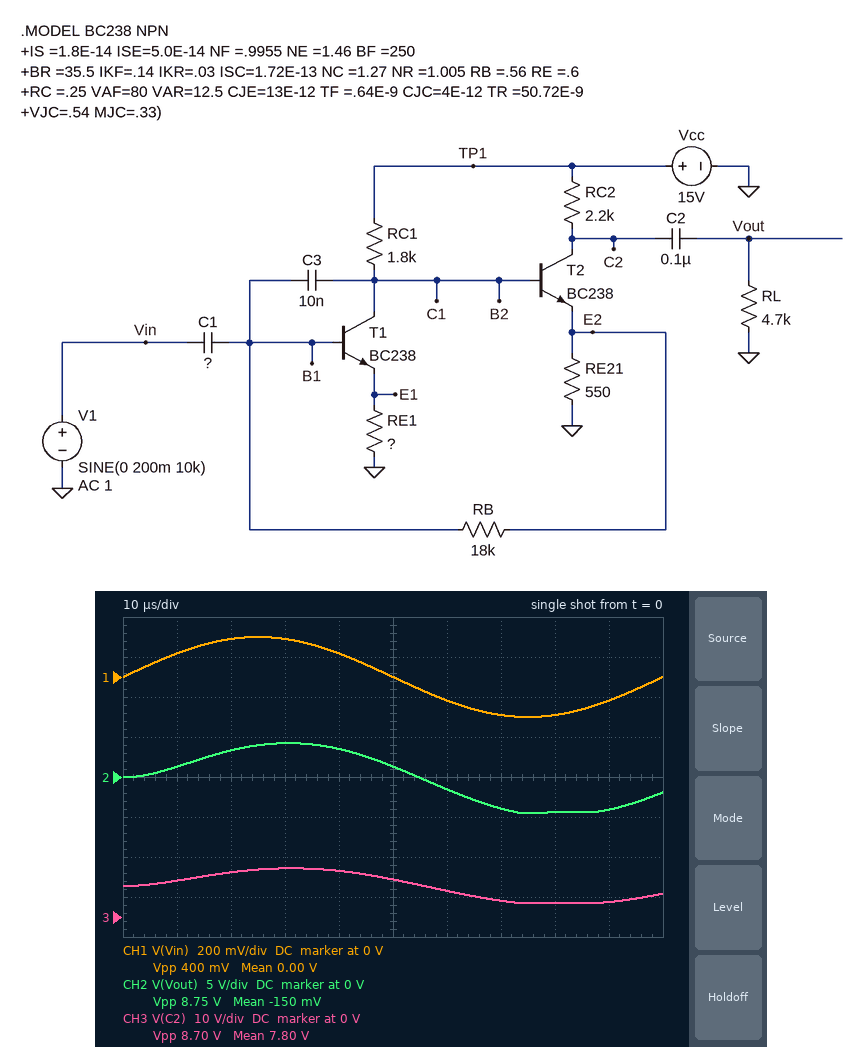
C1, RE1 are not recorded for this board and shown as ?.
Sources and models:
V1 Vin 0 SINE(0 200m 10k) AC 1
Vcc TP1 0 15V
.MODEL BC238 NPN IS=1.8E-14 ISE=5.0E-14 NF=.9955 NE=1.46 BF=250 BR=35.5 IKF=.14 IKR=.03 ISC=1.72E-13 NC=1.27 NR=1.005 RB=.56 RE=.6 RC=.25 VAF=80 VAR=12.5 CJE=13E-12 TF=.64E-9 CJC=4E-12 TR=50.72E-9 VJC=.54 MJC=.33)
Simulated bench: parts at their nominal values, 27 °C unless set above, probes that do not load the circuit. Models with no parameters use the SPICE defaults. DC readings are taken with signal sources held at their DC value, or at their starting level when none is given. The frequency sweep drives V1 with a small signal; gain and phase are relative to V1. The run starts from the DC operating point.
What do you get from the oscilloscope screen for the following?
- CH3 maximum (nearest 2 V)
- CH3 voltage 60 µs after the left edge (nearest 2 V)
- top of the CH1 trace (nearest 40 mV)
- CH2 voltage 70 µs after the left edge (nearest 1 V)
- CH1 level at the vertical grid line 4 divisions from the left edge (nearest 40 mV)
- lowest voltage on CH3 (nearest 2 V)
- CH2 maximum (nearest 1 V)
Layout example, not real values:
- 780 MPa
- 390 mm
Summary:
- 12 V
- 6 V
- 200 mV
- -4 V
- 120 mV
- 4 V
- 4 V
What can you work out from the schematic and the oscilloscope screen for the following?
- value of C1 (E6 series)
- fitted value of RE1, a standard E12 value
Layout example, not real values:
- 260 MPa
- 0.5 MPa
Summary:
- 150 nF
- 68 Ω
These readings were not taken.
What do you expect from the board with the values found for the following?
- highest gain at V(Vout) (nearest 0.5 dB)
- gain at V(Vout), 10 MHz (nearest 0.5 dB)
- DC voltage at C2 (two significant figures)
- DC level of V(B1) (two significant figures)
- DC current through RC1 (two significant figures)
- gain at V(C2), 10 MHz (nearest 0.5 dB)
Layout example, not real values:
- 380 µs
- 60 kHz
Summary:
- 28.0 dB
- 8.5 dB
- 7.8 V
- 1.2 V
- 7.0 mA
- 8.5 dB
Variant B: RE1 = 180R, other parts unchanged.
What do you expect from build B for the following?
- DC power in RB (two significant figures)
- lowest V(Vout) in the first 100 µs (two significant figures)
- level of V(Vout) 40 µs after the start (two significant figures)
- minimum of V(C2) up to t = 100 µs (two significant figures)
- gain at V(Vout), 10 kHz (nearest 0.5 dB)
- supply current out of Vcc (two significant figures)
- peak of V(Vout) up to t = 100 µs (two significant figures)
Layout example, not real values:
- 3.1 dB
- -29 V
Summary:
- 19 µW
- -2.0 V
- 2.4 V
- 3.2 V
- 22.5 dB
- 11 mA
- 2.5 V
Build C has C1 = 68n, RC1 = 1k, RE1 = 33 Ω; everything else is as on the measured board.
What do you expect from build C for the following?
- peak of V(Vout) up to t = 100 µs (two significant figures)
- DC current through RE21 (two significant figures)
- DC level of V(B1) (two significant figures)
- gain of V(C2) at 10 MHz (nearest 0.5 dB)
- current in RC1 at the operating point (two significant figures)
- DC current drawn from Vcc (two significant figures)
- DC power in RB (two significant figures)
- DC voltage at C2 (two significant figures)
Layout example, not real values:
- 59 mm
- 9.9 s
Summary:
- 2.6 V
- 4.0 mA
- 1.1 V
- 8.5 dB
- 12 mA
- 16 mA
- 67 µW
- 6.1 V
